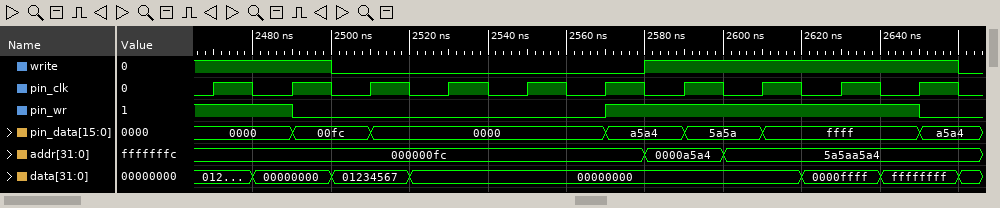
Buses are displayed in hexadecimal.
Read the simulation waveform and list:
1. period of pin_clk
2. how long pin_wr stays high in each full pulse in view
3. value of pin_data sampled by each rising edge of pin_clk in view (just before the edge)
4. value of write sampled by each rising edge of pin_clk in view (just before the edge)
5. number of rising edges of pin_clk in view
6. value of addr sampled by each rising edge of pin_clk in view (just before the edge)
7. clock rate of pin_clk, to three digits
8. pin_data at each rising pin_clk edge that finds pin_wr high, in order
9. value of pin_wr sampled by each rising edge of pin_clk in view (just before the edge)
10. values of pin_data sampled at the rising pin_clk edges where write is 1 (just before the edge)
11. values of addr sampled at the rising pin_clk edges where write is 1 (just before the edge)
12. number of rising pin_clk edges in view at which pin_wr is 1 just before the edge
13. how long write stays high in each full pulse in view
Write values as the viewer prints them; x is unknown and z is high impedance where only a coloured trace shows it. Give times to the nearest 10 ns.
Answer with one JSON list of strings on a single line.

["20 ns", "80 ns", "0000, 0000, 00fc, 0000, 0000, 0000, a5a4, 5a5a, ffff, ffff", "1 1 0 0 0 0 1 1 1 1", "10", "000000fc, 000000fc, 000000fc, 000000fc, 000000fc, 000000fc, 0000a5a4, 5a5aa5a4, 5a5aa5a4, 5a5aa5a4", "50.0 MHz", "0000, 0000, a5a4, 5a5a, ffff, ffff", "1 1 0 0 0 0 1 1 1 1", "0000, 0000, a5a4, 5a5a, ffff, ffff", "000000fc, 000000fc, 0000a5a4, 5a5aa5a4, 5a5aa5a4, 5a5aa5a4", "6", "80 ns"]
